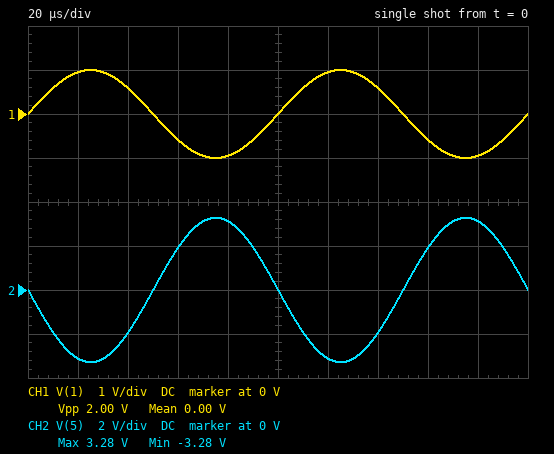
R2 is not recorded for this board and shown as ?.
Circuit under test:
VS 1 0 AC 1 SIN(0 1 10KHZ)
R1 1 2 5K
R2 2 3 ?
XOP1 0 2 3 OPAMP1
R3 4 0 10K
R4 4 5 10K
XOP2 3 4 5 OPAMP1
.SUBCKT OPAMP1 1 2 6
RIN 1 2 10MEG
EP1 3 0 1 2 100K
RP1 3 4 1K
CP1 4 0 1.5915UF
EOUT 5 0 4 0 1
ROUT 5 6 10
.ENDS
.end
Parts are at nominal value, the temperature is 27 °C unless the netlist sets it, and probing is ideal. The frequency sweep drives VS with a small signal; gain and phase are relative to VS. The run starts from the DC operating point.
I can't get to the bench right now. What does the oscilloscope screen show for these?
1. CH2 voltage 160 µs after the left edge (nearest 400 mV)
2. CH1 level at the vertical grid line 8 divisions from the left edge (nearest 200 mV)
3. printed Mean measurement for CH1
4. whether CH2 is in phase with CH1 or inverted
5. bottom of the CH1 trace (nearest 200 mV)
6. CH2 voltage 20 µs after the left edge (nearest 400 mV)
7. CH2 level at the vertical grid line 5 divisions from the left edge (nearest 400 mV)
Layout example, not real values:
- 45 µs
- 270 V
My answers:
- 2.0 V
- -600 mV
- 0.00 V
- inverted
- -1.0 V
- -3.2 V
- 0 V
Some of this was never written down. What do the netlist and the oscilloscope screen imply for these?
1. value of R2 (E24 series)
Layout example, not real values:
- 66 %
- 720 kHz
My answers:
- 8.2 kΩ
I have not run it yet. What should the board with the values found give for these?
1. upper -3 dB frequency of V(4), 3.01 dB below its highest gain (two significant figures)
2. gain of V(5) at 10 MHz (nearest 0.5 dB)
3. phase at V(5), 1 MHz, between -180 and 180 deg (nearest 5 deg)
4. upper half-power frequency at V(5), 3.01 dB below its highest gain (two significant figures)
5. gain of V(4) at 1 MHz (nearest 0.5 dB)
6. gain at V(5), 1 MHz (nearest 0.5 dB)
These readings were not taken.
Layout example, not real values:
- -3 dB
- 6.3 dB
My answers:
- 2.8 MHz
- -5.5 dB
- 155 deg
- 2.8 MHz
- 4.0 dB
- 10.0 dB
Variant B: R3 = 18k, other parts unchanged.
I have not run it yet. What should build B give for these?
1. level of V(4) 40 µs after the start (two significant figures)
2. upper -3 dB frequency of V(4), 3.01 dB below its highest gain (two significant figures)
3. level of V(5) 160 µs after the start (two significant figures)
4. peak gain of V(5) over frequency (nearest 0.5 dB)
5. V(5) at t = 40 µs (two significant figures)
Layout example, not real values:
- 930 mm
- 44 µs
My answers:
- -970 mV
- 3.0 MHz
- 1.5 V
- 8.0 dB
- -1.5 V
